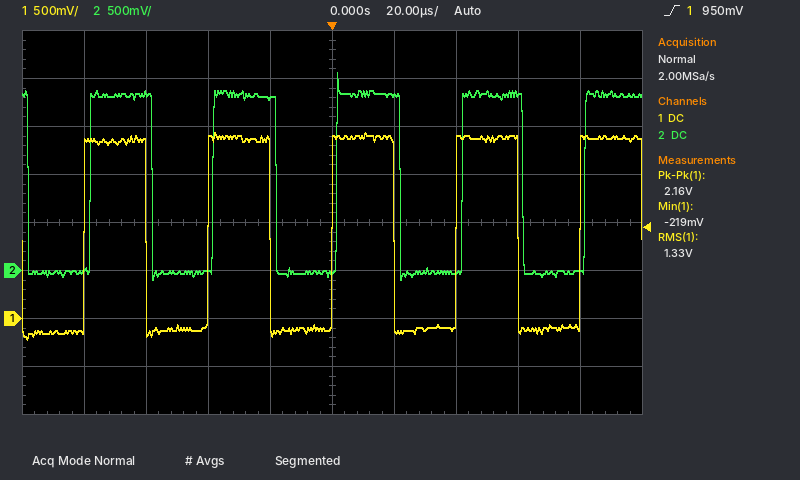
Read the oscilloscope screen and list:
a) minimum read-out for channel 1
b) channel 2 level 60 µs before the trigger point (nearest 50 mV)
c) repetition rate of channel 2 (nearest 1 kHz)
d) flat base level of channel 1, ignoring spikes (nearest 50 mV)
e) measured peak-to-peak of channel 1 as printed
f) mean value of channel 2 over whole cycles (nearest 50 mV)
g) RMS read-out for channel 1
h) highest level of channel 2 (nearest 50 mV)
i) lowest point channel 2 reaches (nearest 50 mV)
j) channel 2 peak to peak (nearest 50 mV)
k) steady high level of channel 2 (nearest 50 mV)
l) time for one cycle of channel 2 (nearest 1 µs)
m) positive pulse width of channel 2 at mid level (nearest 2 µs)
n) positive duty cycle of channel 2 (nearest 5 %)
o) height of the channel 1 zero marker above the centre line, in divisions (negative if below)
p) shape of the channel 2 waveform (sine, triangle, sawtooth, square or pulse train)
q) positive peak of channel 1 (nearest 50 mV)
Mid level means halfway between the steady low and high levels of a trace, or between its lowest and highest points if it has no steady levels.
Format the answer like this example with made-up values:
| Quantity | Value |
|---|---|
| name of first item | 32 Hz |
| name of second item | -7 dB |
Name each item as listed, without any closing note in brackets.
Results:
| Quantity | Value |
|---|---|
| minimum read-out for channel 1 | -219 mV |
| channel 2 level 60 µs before the trigger point | 1.85 V |
| repetition rate of channel 2 | 25 kHz |
| flat base level of channel 1, ignoring spikes | -100 mV |
| measured peak-to-peak of channel 1 as printed | 2.16 V |
| mean value of channel 2 over whole cycles | 900 mV |
| RMS read-out for channel 1 | 1.33 V |
| highest level of channel 2 | 2.05 V |
| lowest point channel 2 reaches | -100 mV |
| channel 2 peak to peak | 2.15 V |
| steady high level of channel 2 | 1.85 V |
| time for one cycle of channel 2 | 40 µs |
| positive pulse width of channel 2 at mid level | 20 µs |
| positive duty cycle of channel 2 | 50 % |
| height of the channel 1 zero marker above the centre line, in divisions | -2.0 div |
| shape of the channel 2 waveform | square |
| positive peak of channel 1 | 1.95 V |
